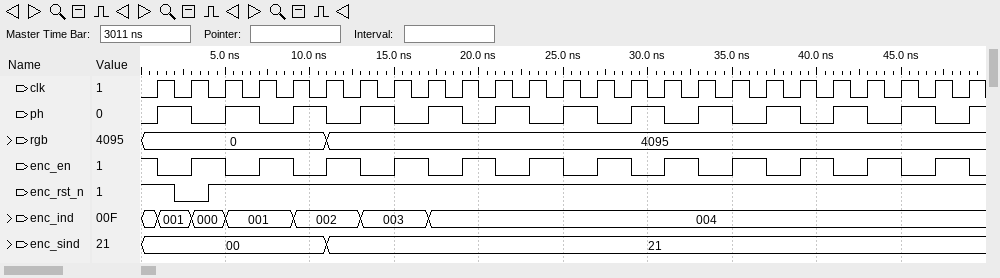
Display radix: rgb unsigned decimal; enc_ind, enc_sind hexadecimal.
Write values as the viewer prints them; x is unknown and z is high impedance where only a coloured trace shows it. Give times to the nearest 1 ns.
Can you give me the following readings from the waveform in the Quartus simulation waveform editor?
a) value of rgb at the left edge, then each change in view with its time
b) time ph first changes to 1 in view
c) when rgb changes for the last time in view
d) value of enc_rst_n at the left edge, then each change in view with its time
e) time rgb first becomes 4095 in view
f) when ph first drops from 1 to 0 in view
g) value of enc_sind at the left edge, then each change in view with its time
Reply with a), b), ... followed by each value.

a) 0, 4095 at 11 ns
b) 1 ns
c) 11 ns
d) 1, 0 at 2 ns, 1 at 4 ns
e) 11 ns
f) 3 ns
g) 00, 21 at 11 ns
